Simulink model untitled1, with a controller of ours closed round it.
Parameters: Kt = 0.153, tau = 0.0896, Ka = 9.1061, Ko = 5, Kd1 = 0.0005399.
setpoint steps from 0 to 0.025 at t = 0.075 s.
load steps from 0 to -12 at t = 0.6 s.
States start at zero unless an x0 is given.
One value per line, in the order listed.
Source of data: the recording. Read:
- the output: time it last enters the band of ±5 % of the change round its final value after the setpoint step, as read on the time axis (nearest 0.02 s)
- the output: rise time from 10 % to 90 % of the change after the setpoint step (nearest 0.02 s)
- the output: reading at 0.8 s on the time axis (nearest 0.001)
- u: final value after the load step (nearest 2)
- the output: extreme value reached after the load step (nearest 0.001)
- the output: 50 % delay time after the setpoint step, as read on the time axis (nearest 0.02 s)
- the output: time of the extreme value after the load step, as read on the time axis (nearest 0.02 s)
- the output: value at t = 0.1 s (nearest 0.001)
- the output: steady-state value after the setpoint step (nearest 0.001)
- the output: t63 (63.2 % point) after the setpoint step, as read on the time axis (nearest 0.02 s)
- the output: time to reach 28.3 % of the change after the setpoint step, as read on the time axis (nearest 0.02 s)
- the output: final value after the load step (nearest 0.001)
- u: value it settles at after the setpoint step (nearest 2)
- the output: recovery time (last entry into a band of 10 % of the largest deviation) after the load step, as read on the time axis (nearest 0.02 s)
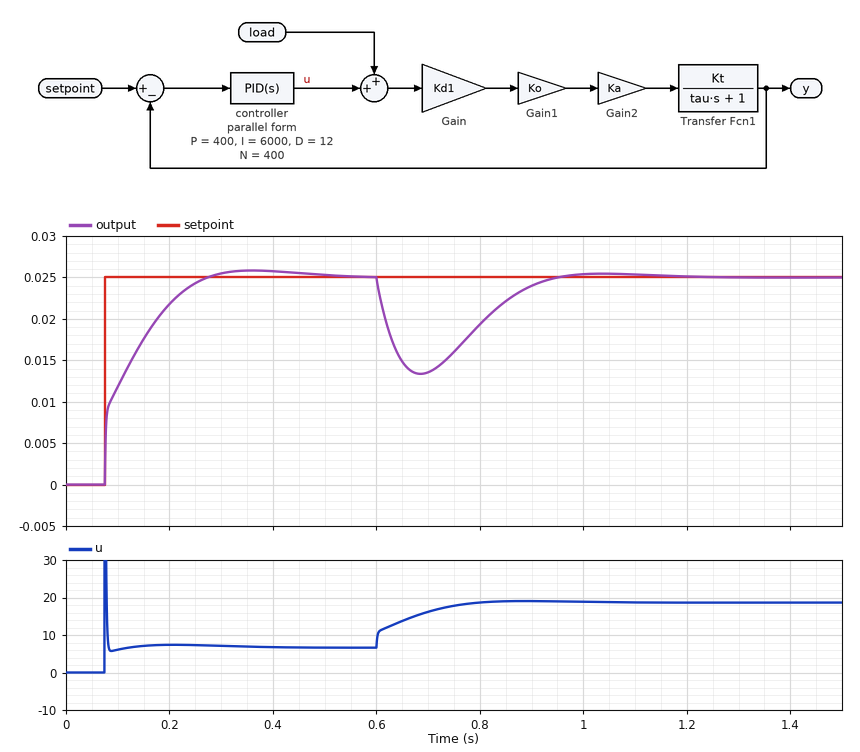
0.24 s
0.14 s
0.019
18
0.013
0.10 s
0.68 s
0.012
0.025
0.14 s
0.08 s
0.025
6
0.90 s
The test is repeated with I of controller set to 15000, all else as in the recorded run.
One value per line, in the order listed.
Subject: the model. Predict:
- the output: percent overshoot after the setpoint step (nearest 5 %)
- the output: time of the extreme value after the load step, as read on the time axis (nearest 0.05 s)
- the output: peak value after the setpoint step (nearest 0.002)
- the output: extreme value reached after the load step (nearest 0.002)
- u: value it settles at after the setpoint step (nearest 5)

15 %
0.65 s
0.028
0.016
5
